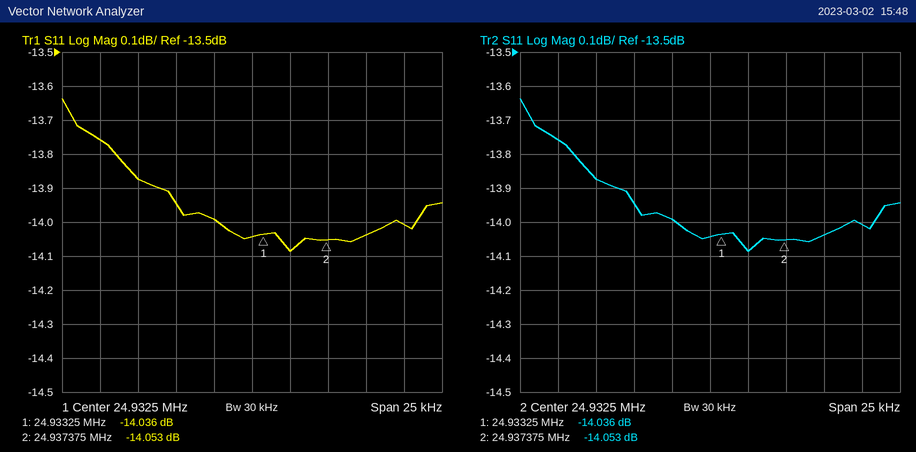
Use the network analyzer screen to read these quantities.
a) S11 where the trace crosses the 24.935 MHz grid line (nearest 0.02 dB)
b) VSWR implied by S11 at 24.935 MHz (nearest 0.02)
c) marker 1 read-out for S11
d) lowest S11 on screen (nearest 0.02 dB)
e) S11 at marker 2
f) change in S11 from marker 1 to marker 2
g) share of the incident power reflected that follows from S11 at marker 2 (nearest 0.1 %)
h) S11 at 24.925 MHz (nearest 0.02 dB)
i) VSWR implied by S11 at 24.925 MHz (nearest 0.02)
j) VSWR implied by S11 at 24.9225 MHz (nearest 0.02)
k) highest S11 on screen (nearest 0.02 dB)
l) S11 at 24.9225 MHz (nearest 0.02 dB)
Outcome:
-14.08 dB
1.50
-14.036 dB
-14.08 dB
-14.053 dB
-0.017 dB
3.9 %
-13.88 dB
1.50
1.52
-13.64 dB
-13.76 dB
